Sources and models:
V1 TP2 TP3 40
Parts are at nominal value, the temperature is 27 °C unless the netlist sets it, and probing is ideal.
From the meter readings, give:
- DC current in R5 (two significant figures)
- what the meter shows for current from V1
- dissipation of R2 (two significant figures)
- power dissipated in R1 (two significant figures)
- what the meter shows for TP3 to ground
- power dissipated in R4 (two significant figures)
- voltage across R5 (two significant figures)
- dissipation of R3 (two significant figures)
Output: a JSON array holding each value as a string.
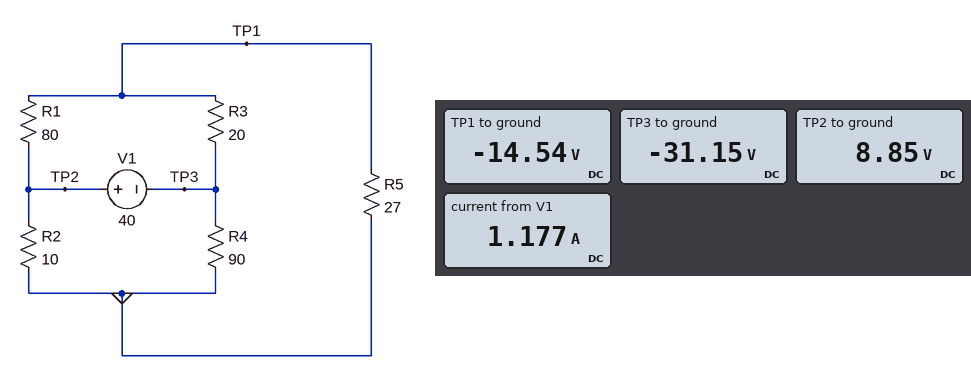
["540 mA", "1.177 A", "7.8 W", "6.8 W", "-31.15 V", "11 W", "15 V", "14 W"]
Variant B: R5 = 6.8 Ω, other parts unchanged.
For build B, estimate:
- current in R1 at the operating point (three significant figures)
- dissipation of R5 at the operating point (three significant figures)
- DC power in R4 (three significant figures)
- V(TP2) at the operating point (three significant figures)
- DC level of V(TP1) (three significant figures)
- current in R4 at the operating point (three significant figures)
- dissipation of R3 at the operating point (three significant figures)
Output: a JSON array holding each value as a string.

["224 mA", "5.27 W", "8.76 W", "11.9 V", "-5.99 V", "312 mA", "24.4 W"]
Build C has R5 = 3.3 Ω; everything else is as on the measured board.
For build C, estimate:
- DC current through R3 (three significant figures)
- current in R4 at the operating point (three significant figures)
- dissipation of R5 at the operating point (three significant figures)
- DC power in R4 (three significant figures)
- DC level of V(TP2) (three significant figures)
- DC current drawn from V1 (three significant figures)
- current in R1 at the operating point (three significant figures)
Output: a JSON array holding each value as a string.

["1.19 A", "301 mA", "3.23 W", "8.16 W", "12.9 V", "1.49 A", "202 mA"]
